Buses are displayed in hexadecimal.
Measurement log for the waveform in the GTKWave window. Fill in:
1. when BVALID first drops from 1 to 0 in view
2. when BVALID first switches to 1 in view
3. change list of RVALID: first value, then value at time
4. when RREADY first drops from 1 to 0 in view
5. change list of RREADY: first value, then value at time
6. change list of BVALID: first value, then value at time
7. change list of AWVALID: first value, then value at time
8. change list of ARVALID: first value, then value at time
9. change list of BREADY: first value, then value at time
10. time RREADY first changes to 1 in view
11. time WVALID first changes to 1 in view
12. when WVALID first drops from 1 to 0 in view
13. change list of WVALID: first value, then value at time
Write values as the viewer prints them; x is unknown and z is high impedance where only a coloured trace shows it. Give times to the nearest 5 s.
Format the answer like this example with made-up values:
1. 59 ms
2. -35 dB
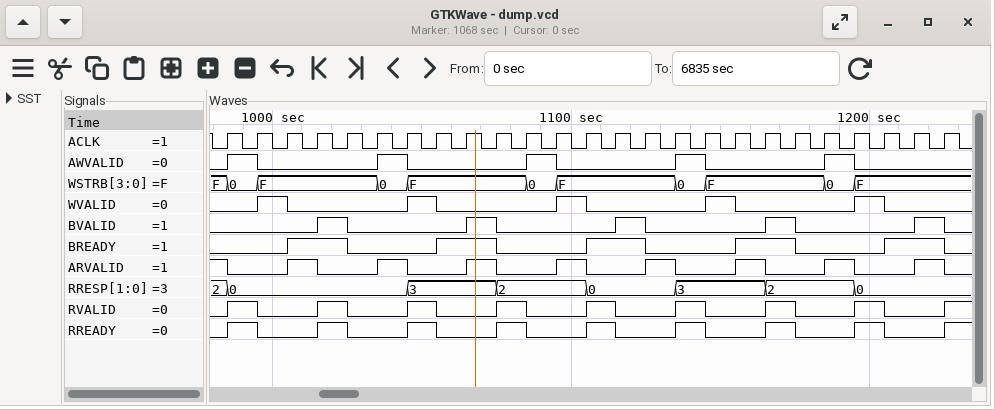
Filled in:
1. 1025 s
2. 1015 s
3. 0, 1 at 985 s, 0 at 995 s, 1 at 1015 s, 0 at 1025 s, 1 at 1045 s, 0 at 1055 s, 1 at 1075 s, 0 at 1085 s, 1 at 1105 s, 0 at 1115 s, 1 at 1135 s, 0 at 1145 s, 1 at 1165 s, 0 at 1175 s, 1 at 1195 s, 0 at 1205 s, 1 at 1225 s
4. 995 s
5. 0, 1 at 985 s, 0 at 995 s, 1 at 1015 s, 0 at 1025 s, 1 at 1045 s, 0 at 1055 s, 1 at 1075 s, 0 at 1085 s, 1 at 1105 s, 0 at 1115 s, 1 at 1135 s, 0 at 1145 s, 1 at 1165 s, 0 at 1175 s, 1 at 1195 s, 0 at 1205 s, 1 at 1225 s
6. 0, 1 at 1015 s, 0 at 1025 s, 1 at 1065 s, 0 at 1075 s, 1 at 1115 s, 0 at 1125 s, 1 at 1165 s, 0 at 1175 s, 1 at 1215 s, 0 at 1225 s
7. 0, 1 at 985 s, 0 at 995 s, 1 at 1035 s, 0 at 1045 s, 1 at 1085 s, 0 at 1095 s, 1 at 1135 s, 0 at 1145 s, 1 at 1185 s, 0 at 1195 s
8. 1, 0 at 985 s, 1 at 1005 s, 0 at 1015 s, 1 at 1035 s, 0 at 1045 s, 1 at 1065 s, 0 at 1075 s, 1 at 1095 s, 0 at 1105 s, 1 at 1125 s, 0 at 1135 s, 1 at 1155 s, 0 at 1165 s, 1 at 1185 s, 0 at 1195 s, 1 at 1215 s, 0 at 1225 s
9. 0, 1 at 1005 s, 0 at 1025 s, 1 at 1055 s, 0 at 1075 s, 1 at 1105 s, 0 at 1125 s, 1 at 1155 s, 0 at 1175 s, 1 at 1205 s, 0 at 1225 s
10. 985 s
11. 995 s
12. 1005 s
13. 0, 1 at 995 s, 0 at 1005 s, 1 at 1045 s, 0 at 1055 s, 1 at 1095 s, 0 at 1105 s, 1 at 1145 s, 0 at 1155 s, 1 at 1195 s, 0 at 1205 s
